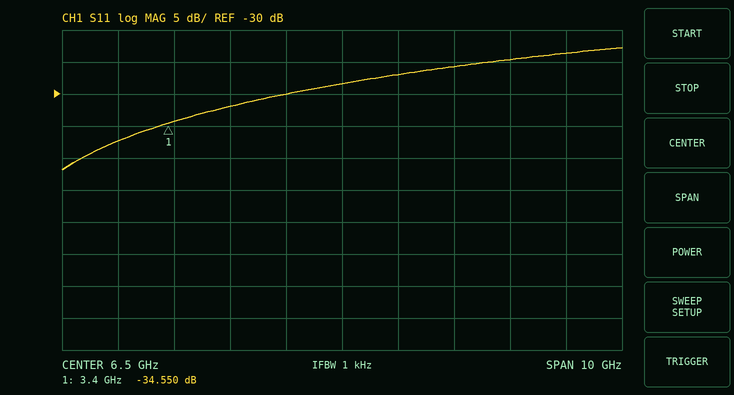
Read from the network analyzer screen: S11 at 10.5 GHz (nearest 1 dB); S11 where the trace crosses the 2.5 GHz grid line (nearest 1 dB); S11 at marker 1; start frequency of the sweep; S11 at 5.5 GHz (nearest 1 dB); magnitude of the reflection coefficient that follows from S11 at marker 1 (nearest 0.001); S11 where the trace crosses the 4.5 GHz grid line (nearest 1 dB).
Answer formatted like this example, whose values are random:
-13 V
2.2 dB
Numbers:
-24 dB
-37 dB
-34.550 dB
1.5 GHz
-30 dB
0.019
-32 dB
